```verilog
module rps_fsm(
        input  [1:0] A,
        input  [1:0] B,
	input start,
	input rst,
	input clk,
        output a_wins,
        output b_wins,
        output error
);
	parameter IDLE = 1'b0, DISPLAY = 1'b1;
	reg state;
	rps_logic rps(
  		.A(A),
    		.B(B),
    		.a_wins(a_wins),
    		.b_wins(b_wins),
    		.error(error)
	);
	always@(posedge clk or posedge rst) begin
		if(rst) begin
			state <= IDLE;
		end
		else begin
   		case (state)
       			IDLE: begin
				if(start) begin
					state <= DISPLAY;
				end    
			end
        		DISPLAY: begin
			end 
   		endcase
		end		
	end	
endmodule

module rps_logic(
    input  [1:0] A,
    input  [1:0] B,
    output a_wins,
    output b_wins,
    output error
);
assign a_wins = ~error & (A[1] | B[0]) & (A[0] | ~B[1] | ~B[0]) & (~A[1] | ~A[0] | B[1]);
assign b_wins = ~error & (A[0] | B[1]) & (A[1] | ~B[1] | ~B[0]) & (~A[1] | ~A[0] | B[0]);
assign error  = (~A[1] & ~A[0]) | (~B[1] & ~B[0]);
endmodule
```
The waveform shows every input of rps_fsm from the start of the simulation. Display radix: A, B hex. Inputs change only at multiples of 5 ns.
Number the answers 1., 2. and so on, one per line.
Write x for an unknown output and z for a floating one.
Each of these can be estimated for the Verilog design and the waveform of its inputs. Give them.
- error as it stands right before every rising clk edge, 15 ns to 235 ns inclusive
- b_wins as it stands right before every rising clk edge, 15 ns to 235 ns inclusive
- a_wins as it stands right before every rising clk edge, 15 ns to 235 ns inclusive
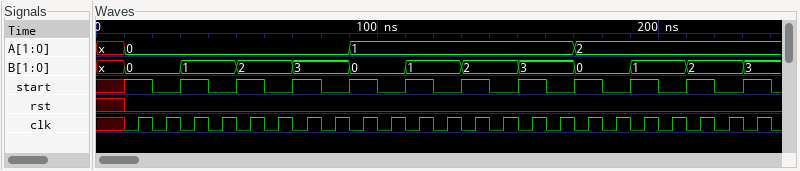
1. 1 1 1 1 1 1 1 1 1 1 0 0 0 0 0 0 1 1 0 0 0 0 0
2. 0 0 0 0 0 0 0 0 0 0 1 1 1 1 0 0 0 0 0 0 1 1 1
3. 0 0 0 0 0 0 0 0 0 0 1 1 0 0 1 1 0 0 1 1 1 1 0
